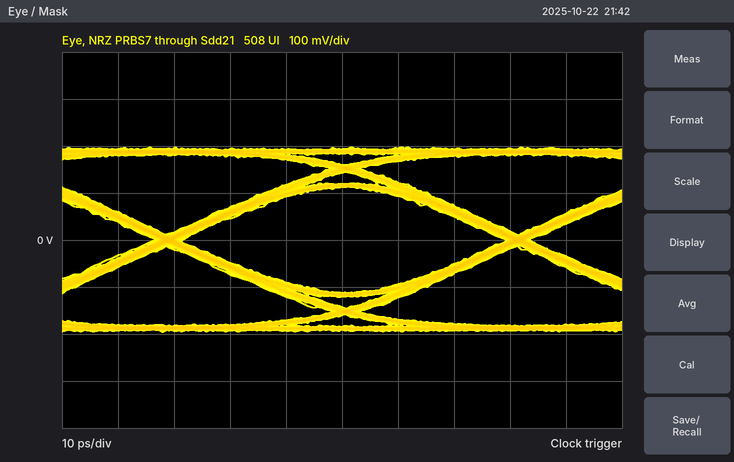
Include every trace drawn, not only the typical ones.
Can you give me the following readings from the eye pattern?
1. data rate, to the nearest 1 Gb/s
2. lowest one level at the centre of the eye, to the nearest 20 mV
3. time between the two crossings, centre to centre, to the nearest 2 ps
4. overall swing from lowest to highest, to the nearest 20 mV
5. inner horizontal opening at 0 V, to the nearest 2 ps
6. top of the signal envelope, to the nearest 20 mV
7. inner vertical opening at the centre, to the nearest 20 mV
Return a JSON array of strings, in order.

["16 Gb/s", "120 mV", "62 ps", "400 mV", "58 ps", "200 mV", "220 mV"]
